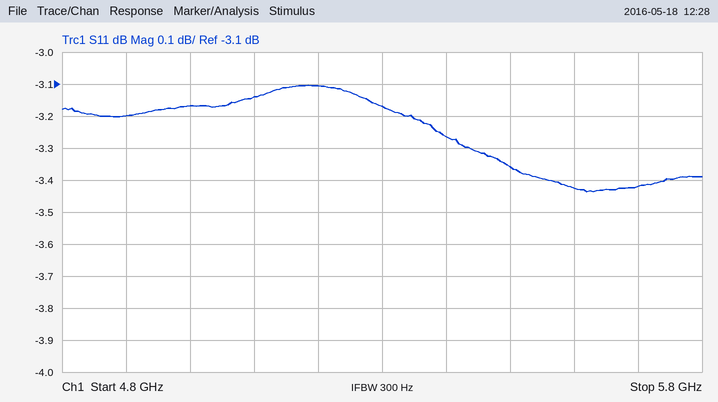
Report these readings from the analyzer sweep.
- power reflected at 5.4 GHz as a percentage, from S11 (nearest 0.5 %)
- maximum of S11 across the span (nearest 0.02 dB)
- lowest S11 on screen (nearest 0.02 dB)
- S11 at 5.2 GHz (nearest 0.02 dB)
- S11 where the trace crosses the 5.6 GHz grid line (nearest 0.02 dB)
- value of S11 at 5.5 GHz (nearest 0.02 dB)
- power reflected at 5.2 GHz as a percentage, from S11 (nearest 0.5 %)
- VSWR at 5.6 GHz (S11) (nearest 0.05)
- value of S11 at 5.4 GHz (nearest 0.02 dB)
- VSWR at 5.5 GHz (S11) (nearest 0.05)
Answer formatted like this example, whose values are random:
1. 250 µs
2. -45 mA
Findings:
1. 47.0 %
2. -3.10 dB
3. -3.44 dB
4. -3.10 dB
5. -3.42 dB
6. -3.36 dB
7. 49.0 %
8. 5.15
9. -3.26 dB
10. 5.25
